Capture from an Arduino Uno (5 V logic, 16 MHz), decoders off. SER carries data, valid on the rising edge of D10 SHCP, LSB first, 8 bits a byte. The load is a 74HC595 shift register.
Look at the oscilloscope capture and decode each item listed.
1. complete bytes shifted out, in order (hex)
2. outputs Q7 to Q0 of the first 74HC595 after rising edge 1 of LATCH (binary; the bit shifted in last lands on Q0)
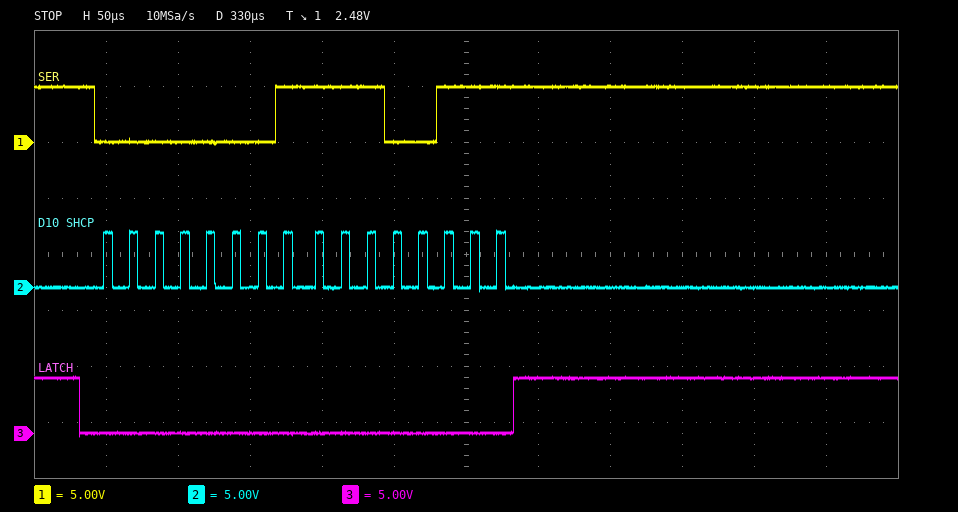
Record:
80 E7
11100111
